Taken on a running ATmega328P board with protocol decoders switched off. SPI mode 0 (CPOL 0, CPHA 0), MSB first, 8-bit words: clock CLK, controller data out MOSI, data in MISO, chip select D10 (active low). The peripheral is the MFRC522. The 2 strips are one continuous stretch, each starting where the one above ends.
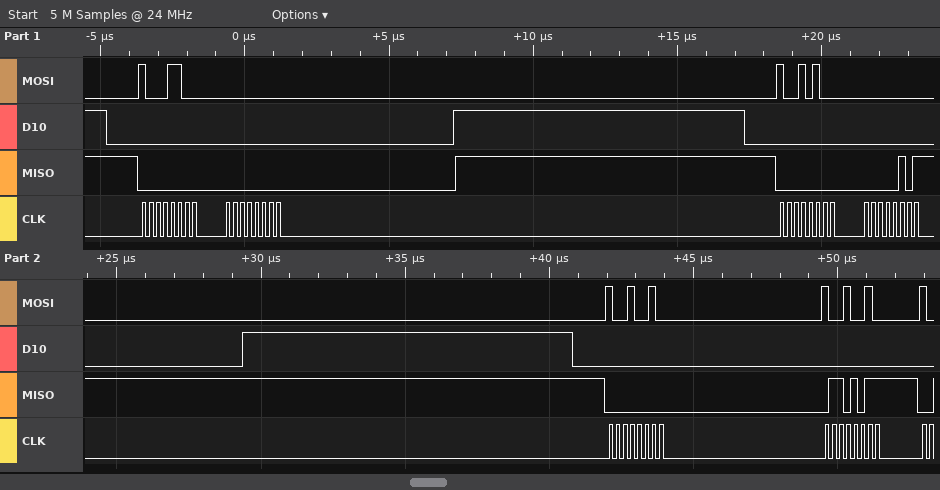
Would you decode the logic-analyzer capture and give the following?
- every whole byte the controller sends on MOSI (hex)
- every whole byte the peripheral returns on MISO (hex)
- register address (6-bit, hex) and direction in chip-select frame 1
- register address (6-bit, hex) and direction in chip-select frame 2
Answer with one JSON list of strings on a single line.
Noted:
["0x8C 0x00 0x94 0x00 0x92 0x92", "0x00 0x00 0x00 0x05 0x00 0x6B", "0x06 read", "0x0A read"]
